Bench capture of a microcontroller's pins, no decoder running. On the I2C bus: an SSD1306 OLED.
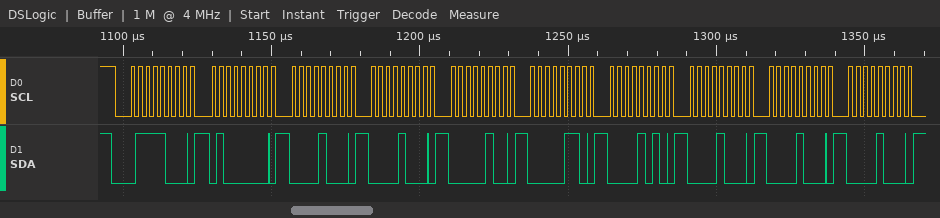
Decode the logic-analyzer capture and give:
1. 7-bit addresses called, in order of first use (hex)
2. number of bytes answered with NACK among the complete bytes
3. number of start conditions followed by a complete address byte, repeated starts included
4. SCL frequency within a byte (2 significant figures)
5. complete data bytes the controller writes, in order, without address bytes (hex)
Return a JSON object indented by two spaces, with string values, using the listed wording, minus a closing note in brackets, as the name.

{
  "7-bit addresses called, in order of first use": "0x3C",
  "number of bytes answered with NACK among the complete bytes": "0",
  "number of start conditions followed by a complete address byte, repeated starts included": "1",
  "SCL frequency within a byte": "400 kHz",
  "complete data bytes the controller writes, in order, without address bytes": "40 08 08 04 06 0A 08 08 08"
}
